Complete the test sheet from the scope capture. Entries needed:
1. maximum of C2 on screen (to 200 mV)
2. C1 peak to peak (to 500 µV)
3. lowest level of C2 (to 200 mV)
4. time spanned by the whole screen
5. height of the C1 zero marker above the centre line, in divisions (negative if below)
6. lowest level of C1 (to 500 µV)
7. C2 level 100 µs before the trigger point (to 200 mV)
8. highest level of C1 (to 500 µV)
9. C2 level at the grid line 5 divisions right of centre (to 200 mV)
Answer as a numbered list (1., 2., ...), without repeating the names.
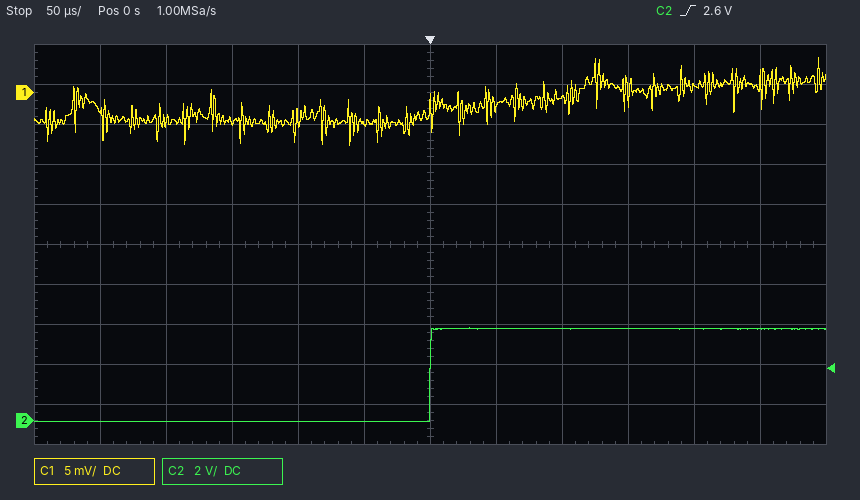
1. 4.6 V
2. 11.0 mV
3. 0.0 V
4. 600 µs
5. +3.8 div
6. -6.5 mV
7. 0.0 V
8. 4.5 mV
9. 4.6 V
